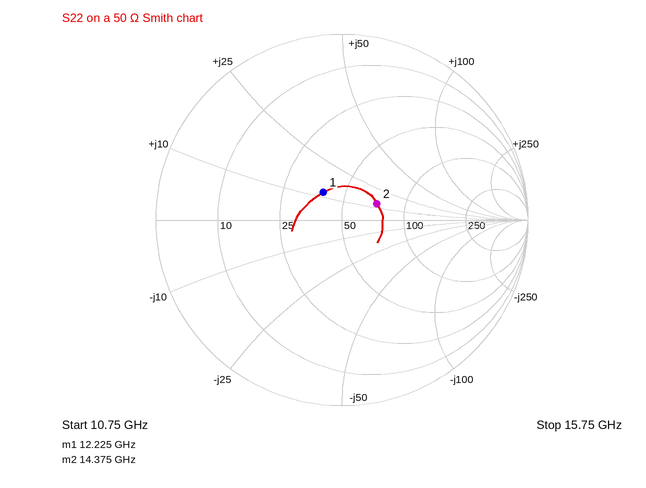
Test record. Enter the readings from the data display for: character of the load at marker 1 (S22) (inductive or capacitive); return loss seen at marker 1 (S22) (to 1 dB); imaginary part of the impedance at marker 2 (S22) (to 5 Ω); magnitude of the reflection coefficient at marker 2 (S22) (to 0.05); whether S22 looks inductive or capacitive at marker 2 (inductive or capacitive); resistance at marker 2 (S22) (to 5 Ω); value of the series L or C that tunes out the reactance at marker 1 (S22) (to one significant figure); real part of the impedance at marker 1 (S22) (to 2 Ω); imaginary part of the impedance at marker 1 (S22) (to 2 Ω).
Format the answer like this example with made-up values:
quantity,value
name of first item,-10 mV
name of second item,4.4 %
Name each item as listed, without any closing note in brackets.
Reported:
quantity,value
character of the load at marker 1 (S22),inductive
return loss seen at marker 1 (S22),15 dB
imaginary part of the impedance at marker 2 (S22),+15 Ω
magnitude of the reflection coefficient at marker 2 (S22),0.20
whether S22 looks inductive or capacitive at marker 2,inductive
resistance at marker 2 (S22),70 Ω
value of the series L or C that tunes out the reactance at marker 1 (S22),1 pF
real part of the impedance at marker 1 (S22),40 Ω
imaginary part of the impedance at marker 1 (S22),+12 Ω
